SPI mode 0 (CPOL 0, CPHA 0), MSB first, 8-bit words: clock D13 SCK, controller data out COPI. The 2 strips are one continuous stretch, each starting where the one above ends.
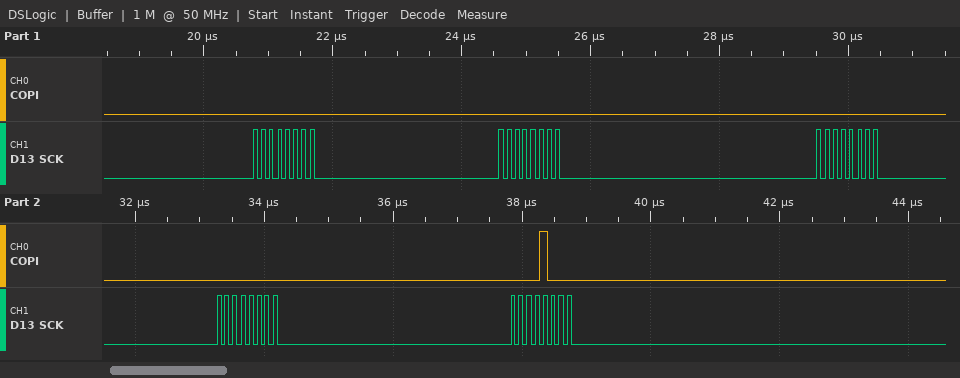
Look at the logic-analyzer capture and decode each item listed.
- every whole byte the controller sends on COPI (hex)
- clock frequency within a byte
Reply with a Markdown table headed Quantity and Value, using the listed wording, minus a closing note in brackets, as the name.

| Quantity | Value |
|---|---|
| every whole byte the controller sends on COPI | 00 00 00 00 08 |
| clock frequency within a byte | 8 MHz |
